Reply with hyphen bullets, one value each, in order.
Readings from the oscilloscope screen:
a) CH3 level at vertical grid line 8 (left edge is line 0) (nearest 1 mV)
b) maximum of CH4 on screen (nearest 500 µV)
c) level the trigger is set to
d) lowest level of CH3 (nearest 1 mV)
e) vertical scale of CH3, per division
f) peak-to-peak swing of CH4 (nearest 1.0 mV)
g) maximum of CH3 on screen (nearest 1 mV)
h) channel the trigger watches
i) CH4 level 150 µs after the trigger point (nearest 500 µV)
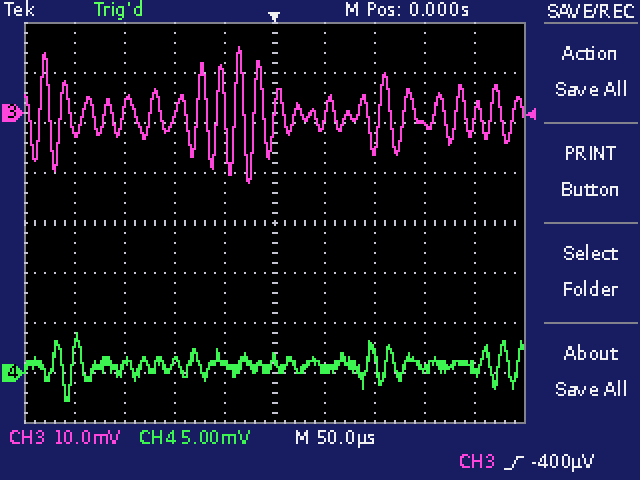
- -2 mV
- 4.0 mV
- -400 µV
- -14 mV
- 10 mV
- 7.0 mV
- 13 mV
- CH3
- 500 µV
